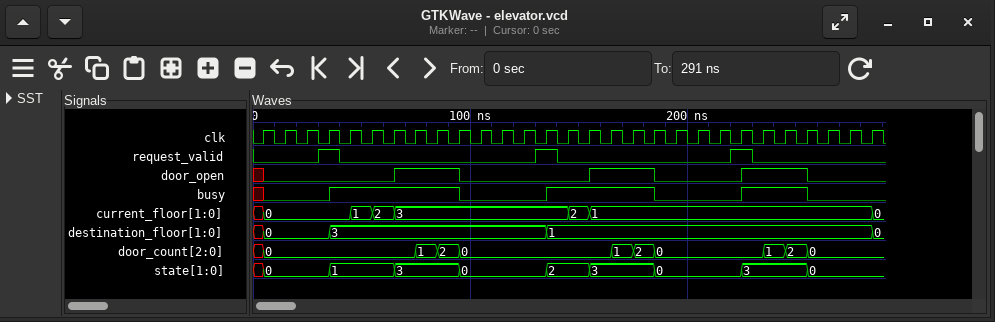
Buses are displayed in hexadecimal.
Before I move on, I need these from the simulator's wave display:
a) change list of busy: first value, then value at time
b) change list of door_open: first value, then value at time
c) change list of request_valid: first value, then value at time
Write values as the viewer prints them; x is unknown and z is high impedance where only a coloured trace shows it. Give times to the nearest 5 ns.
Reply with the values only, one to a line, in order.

x, 0 at 5 ns, 1 at 35 ns, 0 at 95 ns, 1 at 135 ns, 0 at 185 ns, 1 at 225 ns, 0 at 255 ns
x, 0 at 5 ns, 1 at 65 ns, 0 at 95 ns, 1 at 155 ns, 0 at 185 ns, 1 at 225 ns, 0 at 255 ns
0, 1 at 30 ns, 0 at 40 ns, 1 at 130 ns, 0 at 140 ns, 1 at 220 ns, 0 at 230 ns
